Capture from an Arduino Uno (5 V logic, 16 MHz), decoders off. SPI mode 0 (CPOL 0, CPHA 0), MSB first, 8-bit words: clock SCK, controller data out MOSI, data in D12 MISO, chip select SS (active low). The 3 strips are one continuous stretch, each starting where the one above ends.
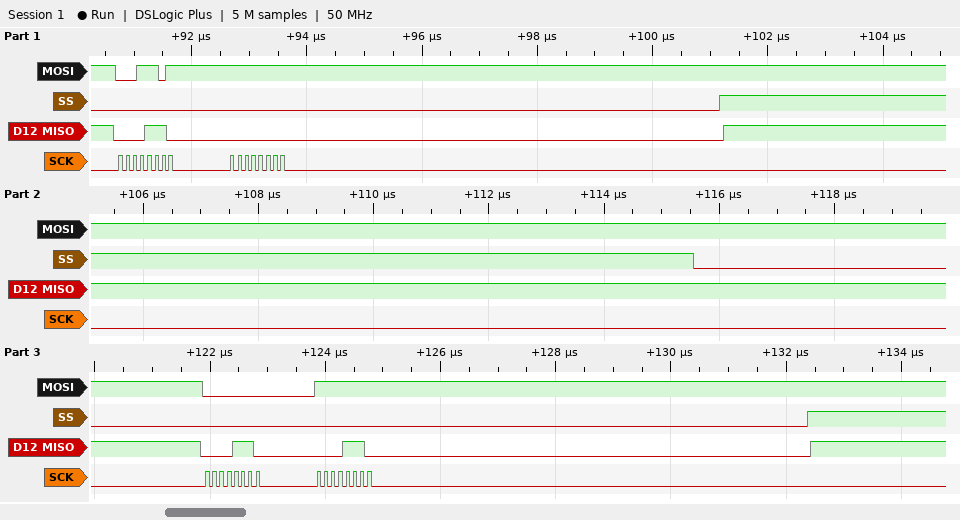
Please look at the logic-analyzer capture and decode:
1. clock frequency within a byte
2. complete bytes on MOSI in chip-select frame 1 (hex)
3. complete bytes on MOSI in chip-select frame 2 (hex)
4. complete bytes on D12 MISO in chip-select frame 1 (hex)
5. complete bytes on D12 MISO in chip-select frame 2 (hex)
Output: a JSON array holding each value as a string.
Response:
["8 MHz", "1D FF", "00 FF", "0E 00", "0E 0E"]
